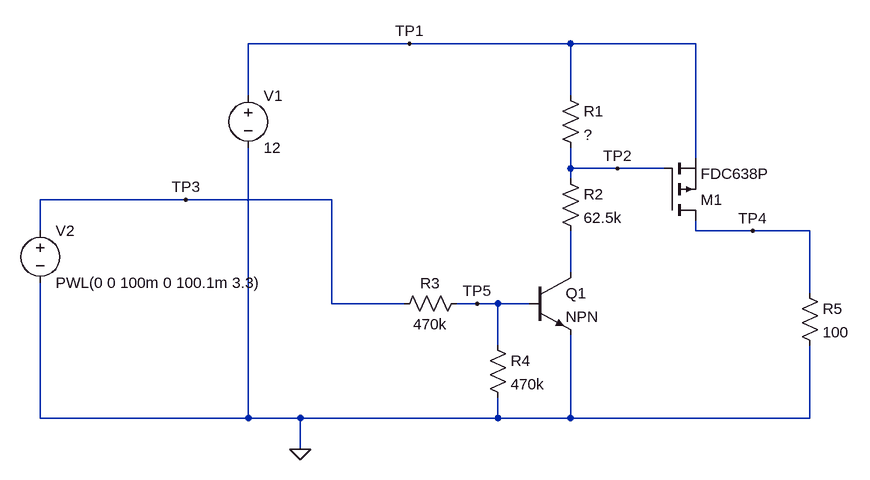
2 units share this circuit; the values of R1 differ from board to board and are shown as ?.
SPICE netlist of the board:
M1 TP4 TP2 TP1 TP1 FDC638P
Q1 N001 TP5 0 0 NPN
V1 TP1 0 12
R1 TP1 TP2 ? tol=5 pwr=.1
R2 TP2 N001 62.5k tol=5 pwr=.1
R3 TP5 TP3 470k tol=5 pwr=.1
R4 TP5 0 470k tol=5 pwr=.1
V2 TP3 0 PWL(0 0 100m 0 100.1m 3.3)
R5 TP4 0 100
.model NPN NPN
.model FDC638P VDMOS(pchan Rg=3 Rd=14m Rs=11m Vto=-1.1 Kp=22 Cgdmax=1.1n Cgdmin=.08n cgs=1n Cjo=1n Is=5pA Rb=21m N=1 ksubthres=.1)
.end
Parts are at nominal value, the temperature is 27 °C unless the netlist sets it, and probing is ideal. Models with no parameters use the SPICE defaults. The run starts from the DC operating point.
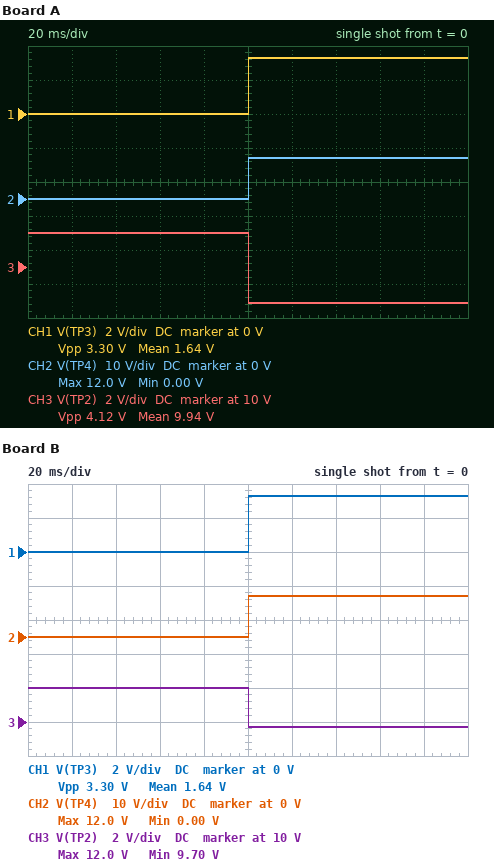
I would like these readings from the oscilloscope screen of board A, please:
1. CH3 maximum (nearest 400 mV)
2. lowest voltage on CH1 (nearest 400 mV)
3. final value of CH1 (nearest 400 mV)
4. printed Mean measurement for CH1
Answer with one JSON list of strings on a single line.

["12.0 V", "0 V", "3.2 V", "1.64 V"]
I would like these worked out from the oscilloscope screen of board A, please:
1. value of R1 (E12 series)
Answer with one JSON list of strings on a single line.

["33 kΩ"]
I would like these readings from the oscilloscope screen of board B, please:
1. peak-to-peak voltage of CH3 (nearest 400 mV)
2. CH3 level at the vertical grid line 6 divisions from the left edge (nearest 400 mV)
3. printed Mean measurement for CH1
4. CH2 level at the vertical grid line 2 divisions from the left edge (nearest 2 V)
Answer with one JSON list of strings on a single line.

["2.4 V", "9.6 V", "1.64 V", "0 V"]
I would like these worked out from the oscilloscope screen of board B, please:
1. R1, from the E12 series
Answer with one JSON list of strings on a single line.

["15 kΩ"]
